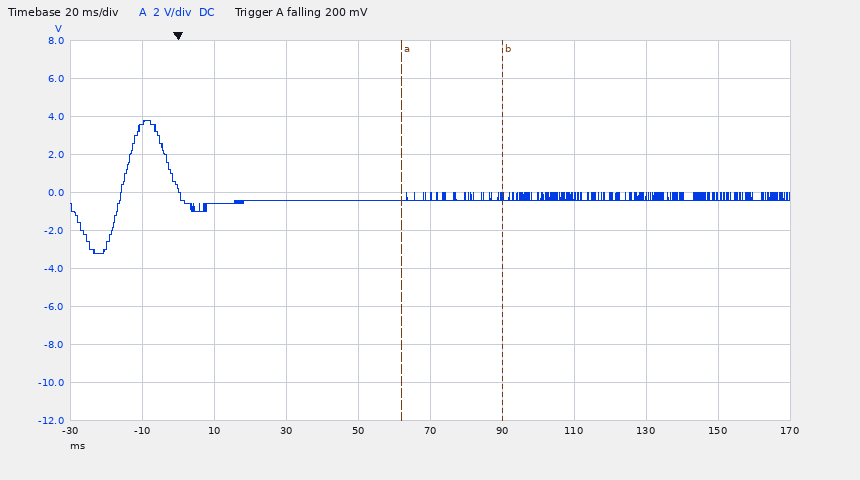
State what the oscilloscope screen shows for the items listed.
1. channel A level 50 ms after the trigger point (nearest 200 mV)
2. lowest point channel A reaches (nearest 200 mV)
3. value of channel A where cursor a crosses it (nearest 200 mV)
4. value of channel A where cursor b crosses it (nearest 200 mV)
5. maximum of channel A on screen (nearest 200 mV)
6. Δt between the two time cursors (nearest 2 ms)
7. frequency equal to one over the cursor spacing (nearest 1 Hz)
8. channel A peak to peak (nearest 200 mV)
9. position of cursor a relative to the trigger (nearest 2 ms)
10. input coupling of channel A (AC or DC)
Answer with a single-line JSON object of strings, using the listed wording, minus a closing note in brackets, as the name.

{"channel A level 50 ms after the trigger point": "-400 mV", "lowest point channel A reaches": "-3.2 V", "value of channel A where cursor a crosses it": "-400 mV", "value of channel A where cursor b crosses it": "-200 mV", "maximum of channel A on screen": "3.8 V", "Δt between the two time cursors": "28 ms", "frequency equal to one over the cursor spacing": "36 Hz", "channel A peak to peak": "7.0 V", "position of cursor a relative to the trigger": "+62 ms", "input coupling of channel A": "DC"}
